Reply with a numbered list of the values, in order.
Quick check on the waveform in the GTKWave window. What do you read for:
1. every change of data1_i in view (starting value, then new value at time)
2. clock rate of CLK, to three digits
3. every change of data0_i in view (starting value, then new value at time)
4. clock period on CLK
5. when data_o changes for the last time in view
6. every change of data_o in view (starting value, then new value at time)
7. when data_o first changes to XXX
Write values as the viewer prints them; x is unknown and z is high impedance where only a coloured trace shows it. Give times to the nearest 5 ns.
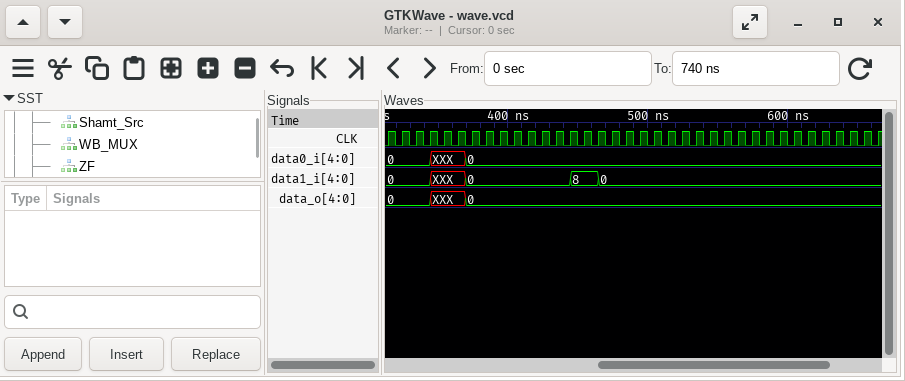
1. 0, XXX at 345 ns, 0 at 370 ns, 8 at 445 ns, 0 at 465 ns
2. 100 MHz
3. 0, XXX at 345 ns, 0 at 370 ns
4. 10 ns
5. 370 ns
6. 0, XXX at 345 ns, 0 at 370 ns
7. 345 ns
